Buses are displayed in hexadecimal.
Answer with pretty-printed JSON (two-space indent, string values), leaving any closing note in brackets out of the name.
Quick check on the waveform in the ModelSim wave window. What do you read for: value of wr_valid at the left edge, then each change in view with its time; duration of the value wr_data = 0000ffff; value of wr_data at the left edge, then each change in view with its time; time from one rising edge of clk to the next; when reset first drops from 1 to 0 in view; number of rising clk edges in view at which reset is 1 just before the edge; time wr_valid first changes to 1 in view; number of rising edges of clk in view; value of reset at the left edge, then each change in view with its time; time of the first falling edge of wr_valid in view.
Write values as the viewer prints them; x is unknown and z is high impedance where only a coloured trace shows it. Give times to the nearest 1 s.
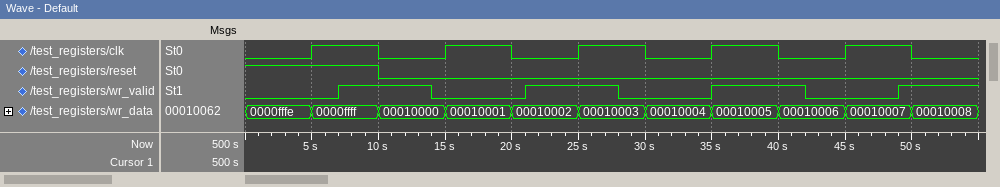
{
  "value of wr_valid at the left edge, then each change in view with its time": "0, 1 at 7 s, 0 at 14 s, 1 at 21 s, 0 at 28 s, 1 at 35 s, 0 at 42 s, 1 at 49 s",
  "duration of the value wr_data = 0000ffff": "5 s",
  "value of wr_data at the left edge, then each change in view with its time": "0000fffe, 0000ffff at 5 s, 00010000 at 10 s, 00010001 at 15 s, 00010002 at 20 s, 00010003 at 25 s, 00010004 at 30 s, 00010005 at 35 s, 00010006 at 40 s, 00010007 at 45 s, 00010008 at 50 s",
  "time from one rising edge of clk to the next": "10 s",
  "when reset first drops from 1 to 0 in view": "10 s",
  "number of rising clk edges in view at which reset is 1 just before the edge": "1",
  "time wr_valid first changes to 1 in view": "7 s",
  "number of rising edges of clk in view": "5",
  "value of reset at the left edge, then each change in view with its time": "1, 0 at 10 s",
  "time of the first falling edge of wr_valid in view": "14 s"
}
